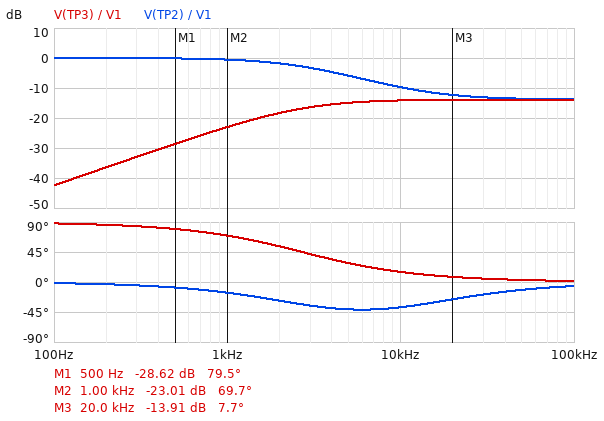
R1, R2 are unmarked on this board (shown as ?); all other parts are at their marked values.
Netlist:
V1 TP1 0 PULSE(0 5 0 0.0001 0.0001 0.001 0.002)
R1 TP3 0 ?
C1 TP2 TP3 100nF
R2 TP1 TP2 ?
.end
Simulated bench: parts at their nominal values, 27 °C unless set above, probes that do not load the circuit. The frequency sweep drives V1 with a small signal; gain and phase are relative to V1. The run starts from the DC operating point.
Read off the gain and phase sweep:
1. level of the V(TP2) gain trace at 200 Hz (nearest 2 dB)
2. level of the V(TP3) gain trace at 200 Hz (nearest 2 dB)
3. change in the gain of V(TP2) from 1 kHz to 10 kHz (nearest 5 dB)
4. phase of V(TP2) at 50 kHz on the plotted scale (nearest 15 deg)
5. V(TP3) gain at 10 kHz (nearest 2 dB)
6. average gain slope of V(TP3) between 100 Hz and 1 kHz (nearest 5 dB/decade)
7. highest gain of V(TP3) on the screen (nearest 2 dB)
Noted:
0 dB
-36 dB
-10 dB
-15 deg
-14 dB
20 dB/decade
-14 dB
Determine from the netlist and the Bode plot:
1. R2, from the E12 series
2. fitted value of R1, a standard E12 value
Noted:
470 Ω
120 Ω
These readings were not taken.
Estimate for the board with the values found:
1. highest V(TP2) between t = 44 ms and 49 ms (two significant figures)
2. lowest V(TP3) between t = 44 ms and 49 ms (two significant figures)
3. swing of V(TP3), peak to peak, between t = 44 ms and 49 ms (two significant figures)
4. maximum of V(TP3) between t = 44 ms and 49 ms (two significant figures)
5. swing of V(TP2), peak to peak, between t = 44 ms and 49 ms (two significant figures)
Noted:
5.0 V
-490 mV
980 mV
490 mV
5.0 V
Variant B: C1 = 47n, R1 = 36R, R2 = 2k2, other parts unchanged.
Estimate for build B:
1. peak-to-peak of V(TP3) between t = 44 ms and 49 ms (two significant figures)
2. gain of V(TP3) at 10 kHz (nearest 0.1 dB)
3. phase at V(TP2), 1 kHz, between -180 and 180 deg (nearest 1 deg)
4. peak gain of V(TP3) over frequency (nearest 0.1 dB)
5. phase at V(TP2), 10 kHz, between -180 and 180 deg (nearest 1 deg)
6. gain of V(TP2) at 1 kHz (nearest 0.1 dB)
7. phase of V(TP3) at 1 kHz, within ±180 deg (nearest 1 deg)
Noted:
100 mV
-36.0 dB
-33 deg
-35.9 dB
-75 deg
-1.6 dB
57 deg
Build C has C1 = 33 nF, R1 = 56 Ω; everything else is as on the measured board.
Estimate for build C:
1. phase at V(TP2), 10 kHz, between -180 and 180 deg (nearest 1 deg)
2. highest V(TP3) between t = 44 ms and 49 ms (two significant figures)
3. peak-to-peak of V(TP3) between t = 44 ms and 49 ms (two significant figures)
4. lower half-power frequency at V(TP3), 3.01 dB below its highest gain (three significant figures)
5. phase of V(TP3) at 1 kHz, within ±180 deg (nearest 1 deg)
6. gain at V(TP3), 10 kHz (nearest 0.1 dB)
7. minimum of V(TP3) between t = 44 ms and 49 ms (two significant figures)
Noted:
-41 deg
92 mV
180 mV
9.17 kHz
84 deg
-22.1 dB
-92 mV
